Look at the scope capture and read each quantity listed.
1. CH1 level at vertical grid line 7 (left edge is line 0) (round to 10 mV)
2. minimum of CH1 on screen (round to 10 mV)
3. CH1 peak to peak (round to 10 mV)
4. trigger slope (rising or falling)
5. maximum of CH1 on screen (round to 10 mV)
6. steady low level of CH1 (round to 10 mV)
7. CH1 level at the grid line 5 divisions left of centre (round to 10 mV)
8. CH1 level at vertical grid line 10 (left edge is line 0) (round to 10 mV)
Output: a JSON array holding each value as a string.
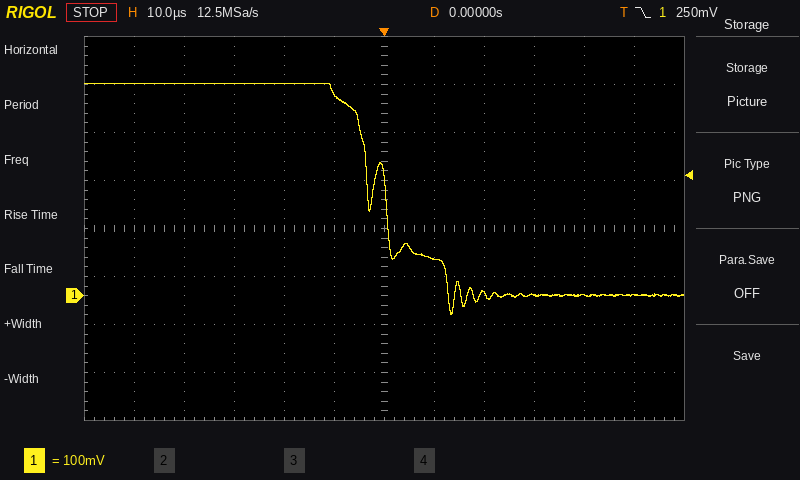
["80 mV", "-40 mV", "480 mV", "falling", "440 mV", "0 mV", "440 mV", "0 mV"]
